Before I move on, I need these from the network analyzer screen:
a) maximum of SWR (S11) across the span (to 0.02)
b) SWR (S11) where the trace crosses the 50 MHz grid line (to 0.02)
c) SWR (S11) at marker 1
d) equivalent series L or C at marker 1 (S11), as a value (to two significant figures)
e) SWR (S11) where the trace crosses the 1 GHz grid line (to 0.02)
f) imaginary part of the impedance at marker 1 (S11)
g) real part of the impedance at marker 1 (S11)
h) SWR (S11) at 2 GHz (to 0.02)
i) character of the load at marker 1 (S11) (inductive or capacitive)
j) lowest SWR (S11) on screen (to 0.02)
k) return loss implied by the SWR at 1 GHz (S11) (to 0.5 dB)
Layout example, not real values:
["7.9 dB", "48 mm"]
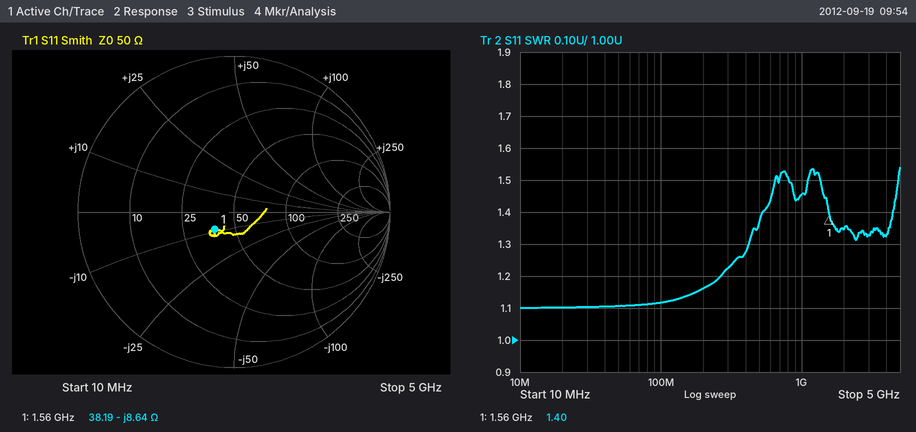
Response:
["1.54", "1.10", "1.40", "12 pF", "1.46", "-8.64 Ω", "38.19 Ω", "1.34", "capacitive", "1.10", "14.5 dB"]
